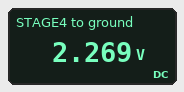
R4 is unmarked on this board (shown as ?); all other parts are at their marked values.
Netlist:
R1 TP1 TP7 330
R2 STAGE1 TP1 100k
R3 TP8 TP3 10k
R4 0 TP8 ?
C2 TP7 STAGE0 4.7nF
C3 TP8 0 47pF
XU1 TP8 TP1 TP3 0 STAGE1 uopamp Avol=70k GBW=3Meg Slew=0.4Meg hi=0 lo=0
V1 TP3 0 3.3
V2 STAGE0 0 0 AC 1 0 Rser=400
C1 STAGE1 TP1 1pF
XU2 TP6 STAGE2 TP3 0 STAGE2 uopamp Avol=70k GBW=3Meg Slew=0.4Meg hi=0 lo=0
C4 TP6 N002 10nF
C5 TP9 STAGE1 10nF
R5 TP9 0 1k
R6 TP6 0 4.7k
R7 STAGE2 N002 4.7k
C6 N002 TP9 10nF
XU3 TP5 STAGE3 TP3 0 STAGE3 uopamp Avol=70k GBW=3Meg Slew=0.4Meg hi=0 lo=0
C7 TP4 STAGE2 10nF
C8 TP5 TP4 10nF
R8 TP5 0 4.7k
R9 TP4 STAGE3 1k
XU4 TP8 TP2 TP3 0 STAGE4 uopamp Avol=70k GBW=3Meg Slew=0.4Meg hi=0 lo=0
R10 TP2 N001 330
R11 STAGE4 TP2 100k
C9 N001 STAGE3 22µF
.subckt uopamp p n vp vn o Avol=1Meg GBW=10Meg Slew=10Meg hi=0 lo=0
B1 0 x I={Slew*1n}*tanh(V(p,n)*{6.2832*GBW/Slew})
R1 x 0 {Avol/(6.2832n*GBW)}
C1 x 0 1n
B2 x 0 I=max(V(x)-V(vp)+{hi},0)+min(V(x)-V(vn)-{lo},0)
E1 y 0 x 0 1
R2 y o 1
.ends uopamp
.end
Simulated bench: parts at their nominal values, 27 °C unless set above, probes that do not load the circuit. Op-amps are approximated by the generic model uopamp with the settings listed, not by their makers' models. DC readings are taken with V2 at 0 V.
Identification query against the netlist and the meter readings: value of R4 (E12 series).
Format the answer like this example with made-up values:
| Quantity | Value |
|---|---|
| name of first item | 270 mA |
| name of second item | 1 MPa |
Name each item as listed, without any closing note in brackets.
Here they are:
| Quantity | Value |
|---|---|
| value of R4 | 22 kΩ |
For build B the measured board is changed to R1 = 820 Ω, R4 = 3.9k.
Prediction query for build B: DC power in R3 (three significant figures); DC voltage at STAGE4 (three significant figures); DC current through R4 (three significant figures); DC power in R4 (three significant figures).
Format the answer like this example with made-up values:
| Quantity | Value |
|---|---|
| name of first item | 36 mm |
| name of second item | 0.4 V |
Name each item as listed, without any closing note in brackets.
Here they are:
| Quantity | Value |
|---|---|
| DC power in R3 | 564 µW |
| DC voltage at STAGE4 | 926 mV |
| DC current through R4 | 237 µA |
| DC power in R4 | 220 µW |
